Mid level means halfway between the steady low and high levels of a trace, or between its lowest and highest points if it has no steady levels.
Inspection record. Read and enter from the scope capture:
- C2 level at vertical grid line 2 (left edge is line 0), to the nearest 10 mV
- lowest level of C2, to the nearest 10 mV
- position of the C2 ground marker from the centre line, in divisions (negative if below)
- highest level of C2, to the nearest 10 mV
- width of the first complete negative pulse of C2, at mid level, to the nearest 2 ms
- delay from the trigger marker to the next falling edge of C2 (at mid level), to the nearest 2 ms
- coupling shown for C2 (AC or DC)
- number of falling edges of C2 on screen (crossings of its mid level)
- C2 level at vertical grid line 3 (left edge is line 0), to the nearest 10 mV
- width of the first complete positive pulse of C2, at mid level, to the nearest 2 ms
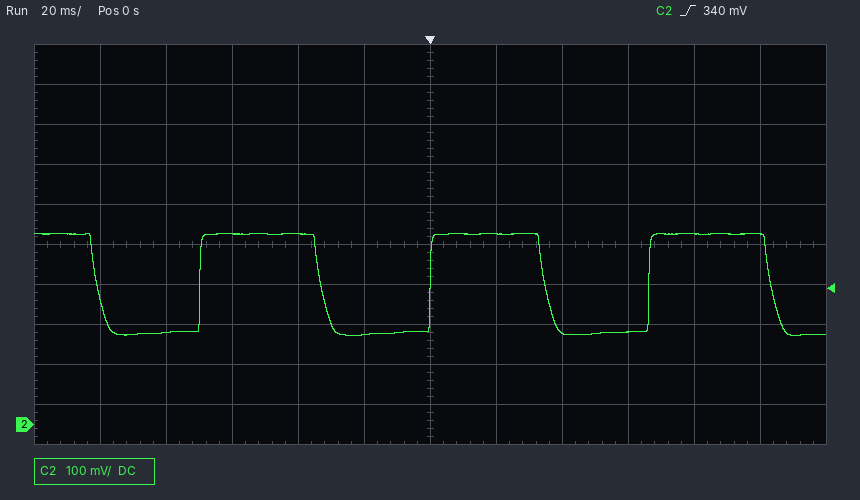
230 mV
220 mV
-4.5 div
480 mV
32 ms
34 ms
DC
4
480 mV
36 ms
